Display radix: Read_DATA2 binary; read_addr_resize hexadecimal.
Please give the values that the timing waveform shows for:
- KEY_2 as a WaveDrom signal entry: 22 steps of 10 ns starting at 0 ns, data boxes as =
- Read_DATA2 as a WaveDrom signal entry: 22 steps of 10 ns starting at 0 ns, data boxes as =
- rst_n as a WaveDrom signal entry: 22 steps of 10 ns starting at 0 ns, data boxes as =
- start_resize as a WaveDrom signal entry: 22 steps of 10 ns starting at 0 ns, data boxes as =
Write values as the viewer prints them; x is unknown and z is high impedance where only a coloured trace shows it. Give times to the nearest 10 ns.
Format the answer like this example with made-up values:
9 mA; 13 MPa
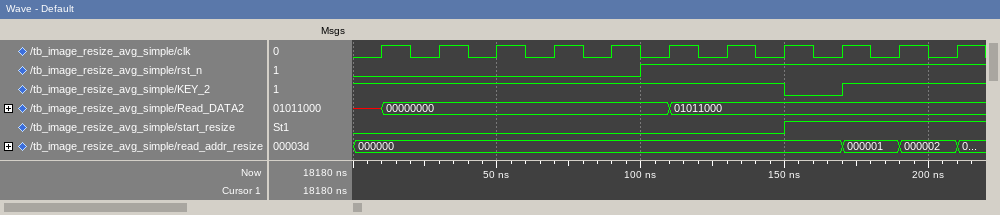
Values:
{name: 'KEY_2', wave: '1..............0.1....'}; {name: 'Read_DATA2', wave: 'x=.........=..........', data: '00000000 01011000'}; {name: 'rst_n', wave: '0.........1...........'}; {name: 'start_resize', wave: '0..............1......'}
